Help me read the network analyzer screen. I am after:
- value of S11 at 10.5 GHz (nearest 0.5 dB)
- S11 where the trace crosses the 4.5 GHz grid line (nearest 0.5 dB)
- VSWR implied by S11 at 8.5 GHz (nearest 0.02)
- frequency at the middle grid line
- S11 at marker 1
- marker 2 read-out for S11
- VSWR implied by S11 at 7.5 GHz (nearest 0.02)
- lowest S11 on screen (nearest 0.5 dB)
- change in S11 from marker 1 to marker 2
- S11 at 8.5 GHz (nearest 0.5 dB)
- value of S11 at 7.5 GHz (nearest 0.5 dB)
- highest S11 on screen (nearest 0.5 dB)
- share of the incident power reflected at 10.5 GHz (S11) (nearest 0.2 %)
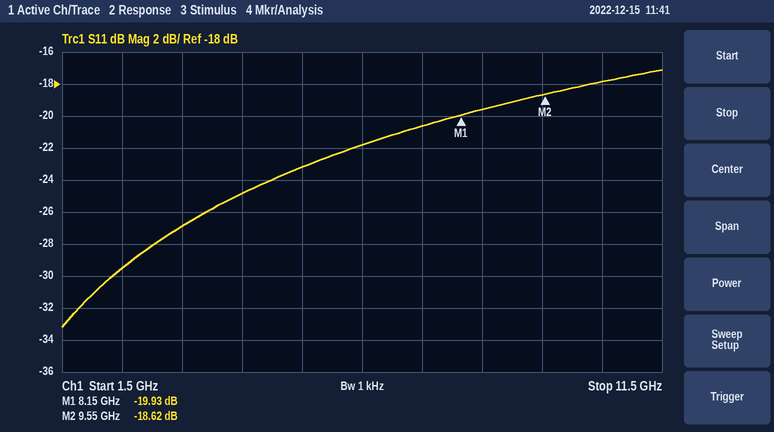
-18.0 dB
-25.0 dB
1.24
6.5 GHz
-19.93 dB
-18.62 dB
1.20
-33.0 dB
1.31 dB
-19.5 dB
-20.5 dB
-17.0 dB
1.6 %
